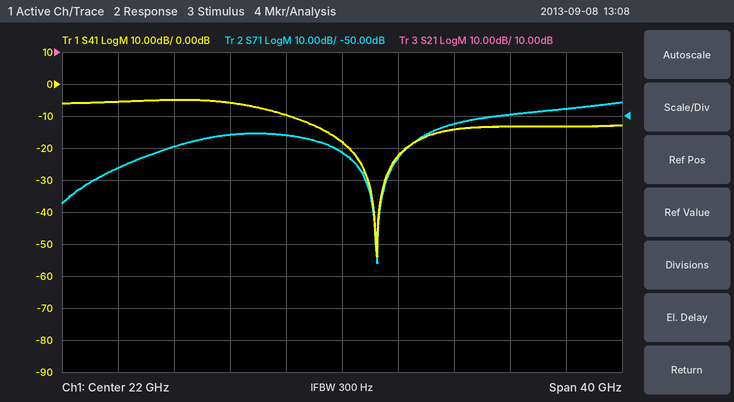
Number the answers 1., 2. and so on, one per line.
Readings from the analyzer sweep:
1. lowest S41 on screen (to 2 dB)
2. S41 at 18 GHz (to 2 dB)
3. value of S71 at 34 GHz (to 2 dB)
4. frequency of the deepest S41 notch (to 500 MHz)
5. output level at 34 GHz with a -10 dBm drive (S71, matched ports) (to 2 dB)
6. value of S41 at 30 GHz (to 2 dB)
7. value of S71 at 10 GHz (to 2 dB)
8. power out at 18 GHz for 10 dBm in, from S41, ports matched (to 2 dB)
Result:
1. -54 dB
2. -10 dB
3. -50 dB
4. 24.5 GHz
5. -60 dBm
6. -14 dB
7. -60 dB
8. 0 dBm
